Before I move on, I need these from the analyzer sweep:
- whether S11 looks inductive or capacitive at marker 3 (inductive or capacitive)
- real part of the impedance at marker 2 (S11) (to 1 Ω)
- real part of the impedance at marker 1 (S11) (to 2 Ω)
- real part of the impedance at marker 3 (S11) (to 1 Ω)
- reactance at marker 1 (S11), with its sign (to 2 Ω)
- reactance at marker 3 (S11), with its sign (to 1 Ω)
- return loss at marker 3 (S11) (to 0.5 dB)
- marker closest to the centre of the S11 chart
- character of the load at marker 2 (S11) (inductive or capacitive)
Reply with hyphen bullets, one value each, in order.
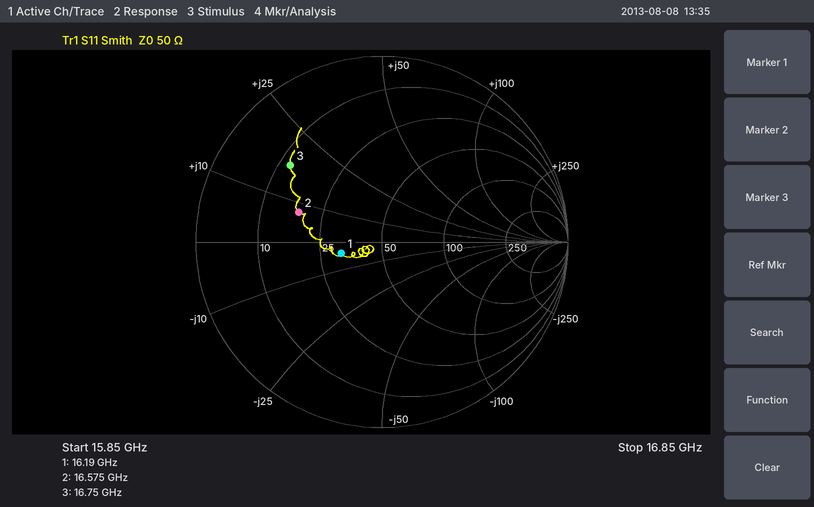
- inductive
- 18 Ω
- 32 Ω
- 12 Ω
- -4 Ω
- +17 Ω
- 4.0 dB
- marker 1
- inductive
